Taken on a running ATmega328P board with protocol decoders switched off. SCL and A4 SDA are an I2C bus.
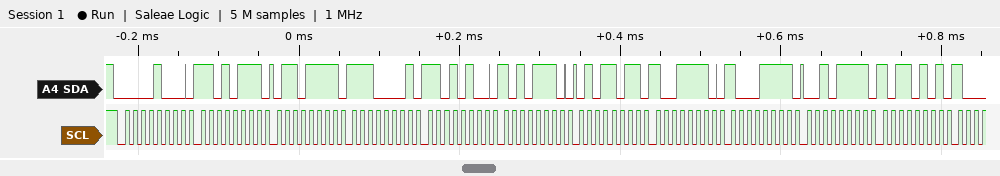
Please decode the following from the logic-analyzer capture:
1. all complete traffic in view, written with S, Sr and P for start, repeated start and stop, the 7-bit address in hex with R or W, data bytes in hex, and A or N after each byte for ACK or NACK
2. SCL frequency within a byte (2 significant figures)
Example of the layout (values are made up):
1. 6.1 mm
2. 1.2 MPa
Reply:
1. S 04W A D7 A 6F A E1 A D4 A AE A 5B A 9E A 8F A 2F A B5 A
2. 100 kHz
